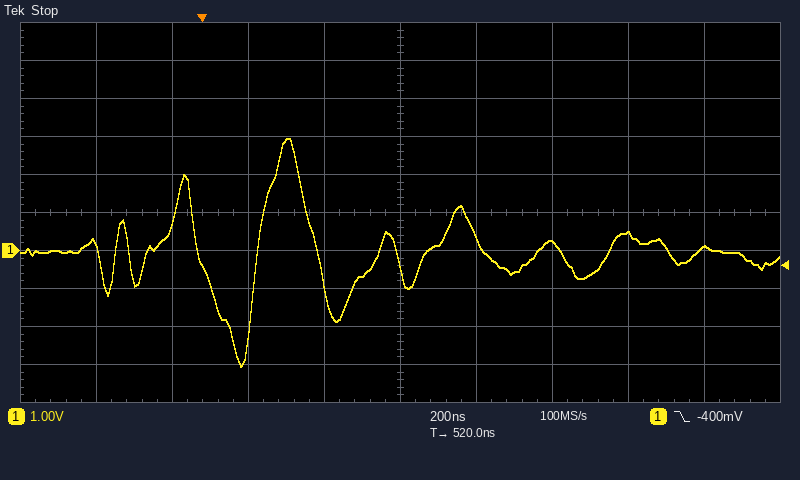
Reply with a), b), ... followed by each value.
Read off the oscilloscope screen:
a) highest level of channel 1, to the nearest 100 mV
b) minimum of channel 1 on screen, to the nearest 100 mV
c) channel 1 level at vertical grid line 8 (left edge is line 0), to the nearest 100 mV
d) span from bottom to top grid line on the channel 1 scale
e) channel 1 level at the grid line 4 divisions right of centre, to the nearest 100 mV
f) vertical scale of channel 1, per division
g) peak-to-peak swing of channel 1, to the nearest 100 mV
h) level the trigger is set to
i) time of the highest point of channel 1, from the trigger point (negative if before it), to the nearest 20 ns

a) 2.9 V
b) -3.1 V
c) 400 mV
d) 10 V
e) 100 mV
f) 1 V
g) 6.0 V
h) -400 mV
i) +220 ns
